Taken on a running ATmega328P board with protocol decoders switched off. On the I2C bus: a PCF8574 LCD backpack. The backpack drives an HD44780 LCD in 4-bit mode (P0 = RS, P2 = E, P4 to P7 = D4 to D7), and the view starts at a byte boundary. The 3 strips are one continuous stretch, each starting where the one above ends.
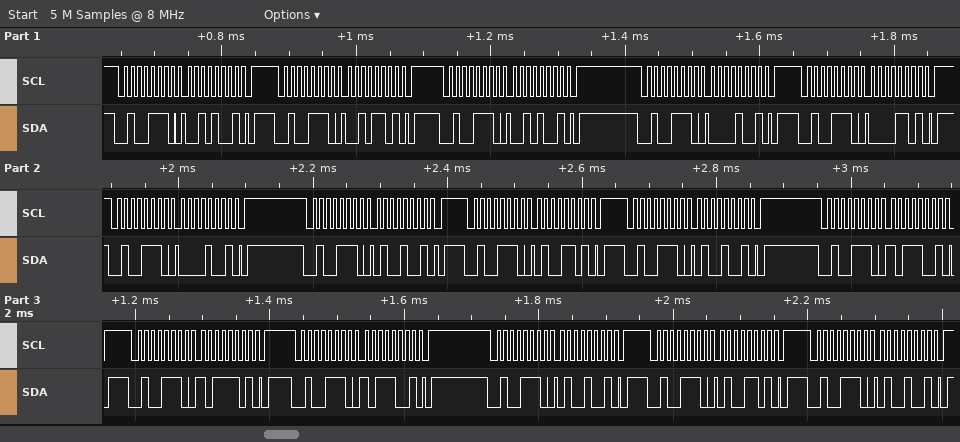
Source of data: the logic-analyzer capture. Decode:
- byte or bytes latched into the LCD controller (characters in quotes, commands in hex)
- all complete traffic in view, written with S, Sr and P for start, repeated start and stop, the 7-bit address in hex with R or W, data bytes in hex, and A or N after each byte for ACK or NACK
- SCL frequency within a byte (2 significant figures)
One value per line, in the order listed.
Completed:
' ' 'K'
S 27W A 29 A P S 27W A 2D A P S 27W A 29 A P S 27W A 09 A P S 27W A 0D A P S 27W A 09 A P S 27W A 49 A P S 27W A 4D A P S 27W A 49 A P S 27W A B9 A P S 27W A BD A P S 27W A B9 A P S 27W A 49 A P S 27W A 4D A P S 27W A 49 A P
100 kHz
